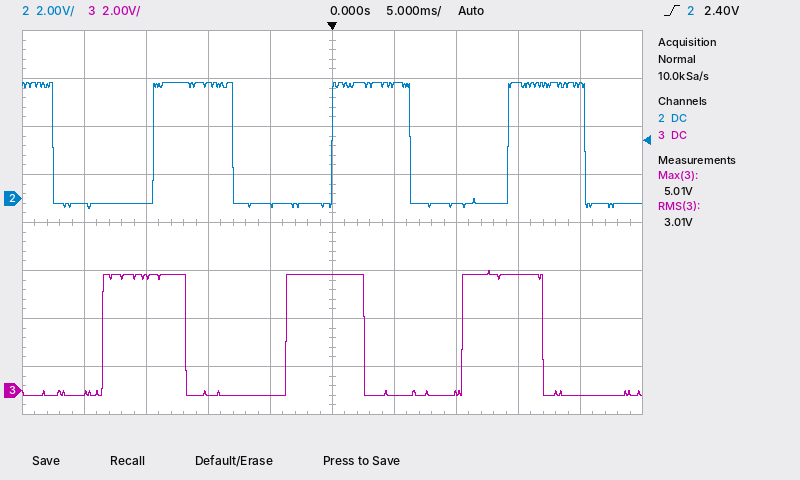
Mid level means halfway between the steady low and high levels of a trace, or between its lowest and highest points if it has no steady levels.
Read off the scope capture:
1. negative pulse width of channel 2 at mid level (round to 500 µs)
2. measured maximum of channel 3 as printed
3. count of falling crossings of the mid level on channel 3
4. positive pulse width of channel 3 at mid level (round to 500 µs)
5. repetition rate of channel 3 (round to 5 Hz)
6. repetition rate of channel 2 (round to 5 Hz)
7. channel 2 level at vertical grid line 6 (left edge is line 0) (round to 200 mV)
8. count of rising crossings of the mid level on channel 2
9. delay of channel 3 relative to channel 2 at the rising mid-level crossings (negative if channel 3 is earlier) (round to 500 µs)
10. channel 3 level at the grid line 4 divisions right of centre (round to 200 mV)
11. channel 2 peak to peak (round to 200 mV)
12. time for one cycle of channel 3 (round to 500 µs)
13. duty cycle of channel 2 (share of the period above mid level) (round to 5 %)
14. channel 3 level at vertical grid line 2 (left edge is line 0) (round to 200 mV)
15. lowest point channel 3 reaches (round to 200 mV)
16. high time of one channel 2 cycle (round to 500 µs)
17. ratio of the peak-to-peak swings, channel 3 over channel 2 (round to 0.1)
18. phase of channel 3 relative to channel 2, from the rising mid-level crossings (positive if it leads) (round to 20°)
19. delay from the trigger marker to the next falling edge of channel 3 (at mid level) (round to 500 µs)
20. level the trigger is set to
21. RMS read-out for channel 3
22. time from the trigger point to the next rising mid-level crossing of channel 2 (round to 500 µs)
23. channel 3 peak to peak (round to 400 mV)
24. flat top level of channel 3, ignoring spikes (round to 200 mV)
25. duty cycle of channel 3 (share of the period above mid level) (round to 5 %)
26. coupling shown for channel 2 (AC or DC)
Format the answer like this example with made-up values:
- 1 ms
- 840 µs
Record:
- 8.0 ms
- 5.01 V
- 3
- 6.5 ms
- 70 Hz
- 70 Hz
- 4.8 V
- 3
- -4.0 ms
- -200 mV
- 5.2 V
- 14.5 ms
- 45 %
- 4.8 V
- -200 mV
- 6.5 ms
- 1.0
- +100°
- 2.5 ms
- 2.40 V
- 3.01 V
- 14.0 ms
- 5.2 V
- 4.8 V
- 45 %
- DC
